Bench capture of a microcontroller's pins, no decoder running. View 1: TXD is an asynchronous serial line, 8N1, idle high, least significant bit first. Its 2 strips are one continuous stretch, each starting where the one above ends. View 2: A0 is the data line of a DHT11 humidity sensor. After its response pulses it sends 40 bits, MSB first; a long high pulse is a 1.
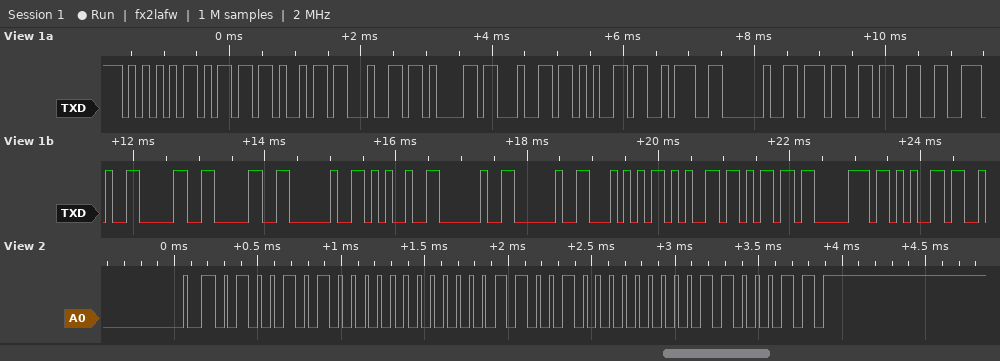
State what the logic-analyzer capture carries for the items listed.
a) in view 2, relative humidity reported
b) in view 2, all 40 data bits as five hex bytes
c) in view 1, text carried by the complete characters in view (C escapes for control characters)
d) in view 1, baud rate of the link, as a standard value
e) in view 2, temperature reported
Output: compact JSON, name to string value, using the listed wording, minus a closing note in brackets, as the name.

{"in view 2, relative humidity reported": "74 %", "in view 2, all 40 data bits as five hex bytes": "4A 00 19 00 63", "in view 1, text carried by the complete characters in view": "\"Umidade: 73.00 %  Tempe\"", "in view 1, baud rate of the link, as a standard value": "9600 baud", "in view 2, temperature reported": "25.0 °C"}
